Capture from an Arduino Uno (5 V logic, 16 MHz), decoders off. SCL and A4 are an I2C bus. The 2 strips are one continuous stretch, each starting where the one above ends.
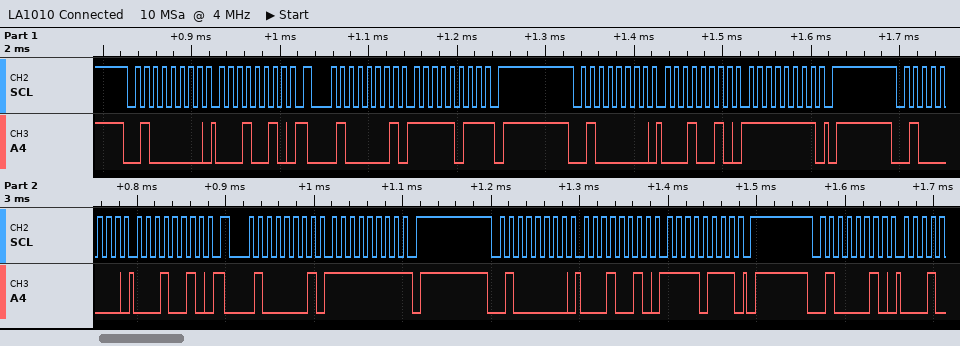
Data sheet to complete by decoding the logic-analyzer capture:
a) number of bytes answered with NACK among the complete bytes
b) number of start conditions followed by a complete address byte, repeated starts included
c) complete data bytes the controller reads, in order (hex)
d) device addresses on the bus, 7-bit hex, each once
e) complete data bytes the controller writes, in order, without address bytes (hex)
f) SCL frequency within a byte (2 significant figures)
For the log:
2
7
FB FF
0x20 0x21
12 12 FF 12 12 F7
100 kHz
